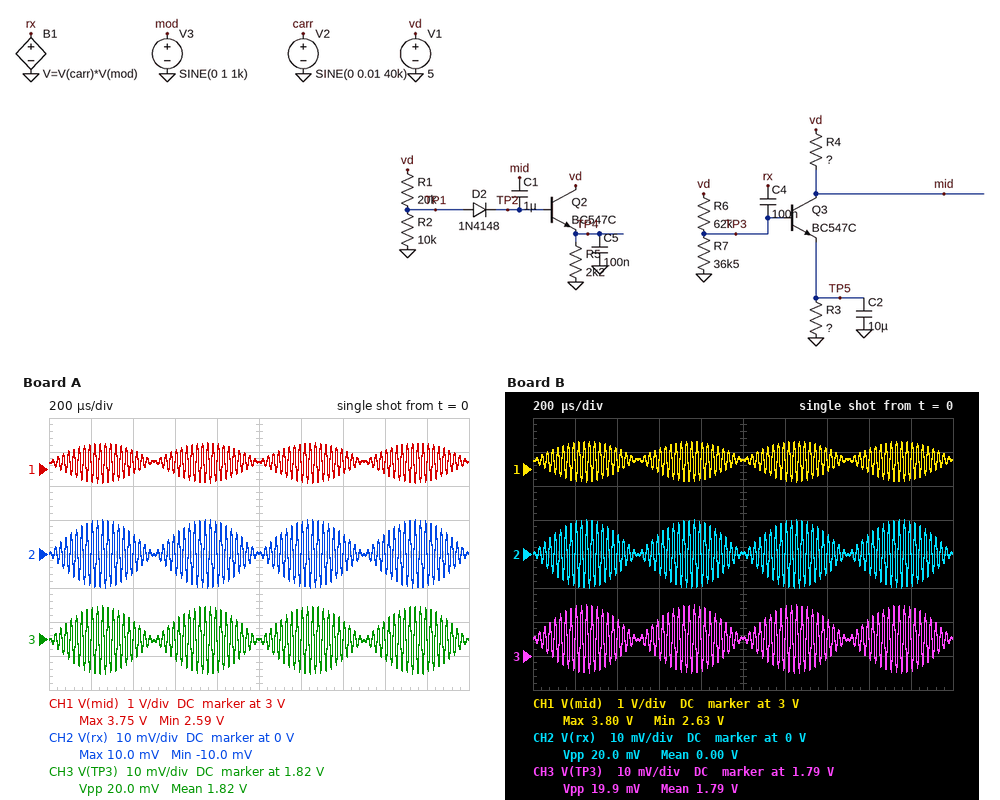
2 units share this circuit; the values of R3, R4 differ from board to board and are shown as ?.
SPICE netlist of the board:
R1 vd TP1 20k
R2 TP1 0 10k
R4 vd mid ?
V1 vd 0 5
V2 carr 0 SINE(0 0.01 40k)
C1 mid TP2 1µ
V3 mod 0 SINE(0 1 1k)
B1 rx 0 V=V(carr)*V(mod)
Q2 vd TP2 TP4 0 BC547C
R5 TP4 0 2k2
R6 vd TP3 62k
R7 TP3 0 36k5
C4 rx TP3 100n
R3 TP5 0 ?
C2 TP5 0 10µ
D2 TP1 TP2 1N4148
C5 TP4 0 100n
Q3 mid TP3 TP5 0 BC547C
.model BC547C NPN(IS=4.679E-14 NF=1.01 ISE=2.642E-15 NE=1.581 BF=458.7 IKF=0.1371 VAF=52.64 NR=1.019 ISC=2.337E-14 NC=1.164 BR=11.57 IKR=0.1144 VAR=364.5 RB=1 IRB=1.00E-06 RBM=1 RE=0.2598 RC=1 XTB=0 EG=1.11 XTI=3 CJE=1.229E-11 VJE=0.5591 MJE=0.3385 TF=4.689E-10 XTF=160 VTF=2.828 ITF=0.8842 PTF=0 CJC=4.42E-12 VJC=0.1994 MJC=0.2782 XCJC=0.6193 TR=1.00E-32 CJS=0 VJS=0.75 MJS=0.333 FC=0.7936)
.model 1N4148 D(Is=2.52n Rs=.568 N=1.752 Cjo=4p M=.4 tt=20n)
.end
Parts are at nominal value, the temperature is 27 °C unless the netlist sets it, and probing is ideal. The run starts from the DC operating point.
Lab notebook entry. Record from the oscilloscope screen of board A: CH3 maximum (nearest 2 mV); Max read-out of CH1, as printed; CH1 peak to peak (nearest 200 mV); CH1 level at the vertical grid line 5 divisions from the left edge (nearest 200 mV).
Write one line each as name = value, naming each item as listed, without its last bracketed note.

CH3 maximum = 1.830 V
Max read-out of CH1, as printed = 3.75 V
CH1 peak to peak = 1.2 V
CH1 level at the vertical grid line 5 divisions from the left edge = 3.2 V
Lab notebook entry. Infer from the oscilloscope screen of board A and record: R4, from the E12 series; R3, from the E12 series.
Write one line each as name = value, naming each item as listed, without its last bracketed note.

R4, from the E12 series = 2.7 kΩ
R3, from the E12 series = 1.8 kΩ
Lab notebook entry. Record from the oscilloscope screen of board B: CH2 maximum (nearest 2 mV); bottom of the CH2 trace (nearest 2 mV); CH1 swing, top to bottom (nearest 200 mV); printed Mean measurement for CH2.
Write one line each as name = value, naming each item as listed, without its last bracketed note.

CH2 maximum = 10 mV
bottom of the CH2 trace = -10 mV
CH1 swing, top to bottom = 1.2 V
printed Mean measurement for CH2 = 0.00 V
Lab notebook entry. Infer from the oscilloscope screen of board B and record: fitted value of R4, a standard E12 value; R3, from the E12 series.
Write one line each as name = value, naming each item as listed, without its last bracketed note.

fitted value of R4, a standard E12 value = 1.5 kΩ
R3, from the E12 series = 1 kΩ
